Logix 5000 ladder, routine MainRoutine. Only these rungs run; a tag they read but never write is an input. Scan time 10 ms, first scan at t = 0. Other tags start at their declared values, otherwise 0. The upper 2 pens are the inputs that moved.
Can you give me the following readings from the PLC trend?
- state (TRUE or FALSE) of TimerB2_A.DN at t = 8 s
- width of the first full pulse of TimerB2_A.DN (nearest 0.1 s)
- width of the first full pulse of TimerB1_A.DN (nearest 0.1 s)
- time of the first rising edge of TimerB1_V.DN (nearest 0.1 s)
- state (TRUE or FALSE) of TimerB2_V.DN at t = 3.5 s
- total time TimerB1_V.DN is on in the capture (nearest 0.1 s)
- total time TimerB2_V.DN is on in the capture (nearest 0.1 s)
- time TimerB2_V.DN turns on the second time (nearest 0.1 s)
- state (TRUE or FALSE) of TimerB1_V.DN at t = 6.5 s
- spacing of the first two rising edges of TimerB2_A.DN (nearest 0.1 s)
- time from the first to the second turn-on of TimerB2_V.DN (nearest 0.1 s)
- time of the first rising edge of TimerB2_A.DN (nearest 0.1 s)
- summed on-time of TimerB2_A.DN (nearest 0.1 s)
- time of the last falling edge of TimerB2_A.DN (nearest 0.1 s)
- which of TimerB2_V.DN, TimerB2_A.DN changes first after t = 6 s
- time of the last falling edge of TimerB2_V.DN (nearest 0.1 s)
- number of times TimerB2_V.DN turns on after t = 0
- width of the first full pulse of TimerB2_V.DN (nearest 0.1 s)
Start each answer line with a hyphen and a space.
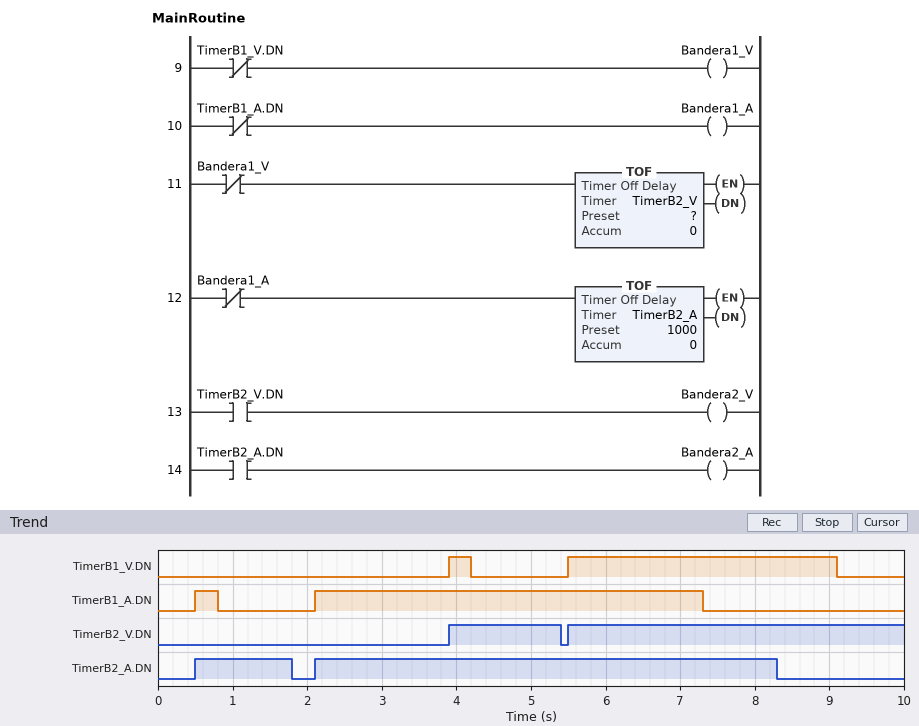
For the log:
- TRUE
- 1.3 s
- 0.3 s
- 3.9 s
- FALSE
- 3.9 s
- 6.0 s
- 5.5 s
- TRUE
- 1.6 s
- 1.6 s
- 0.5 s
- 7.5 s
- 8.3 s
- TimerB2_A.DN
- 5.4 s
- 2
- 1.5 s
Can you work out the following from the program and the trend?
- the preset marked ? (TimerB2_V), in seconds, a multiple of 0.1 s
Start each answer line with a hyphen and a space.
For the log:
- 1.2 s
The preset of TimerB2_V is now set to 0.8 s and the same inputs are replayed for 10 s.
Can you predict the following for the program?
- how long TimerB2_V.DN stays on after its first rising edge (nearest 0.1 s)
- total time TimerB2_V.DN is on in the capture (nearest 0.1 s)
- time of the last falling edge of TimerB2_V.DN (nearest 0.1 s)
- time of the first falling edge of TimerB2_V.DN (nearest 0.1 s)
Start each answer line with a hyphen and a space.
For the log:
- 1.1 s
- 5.5 s
- 9.9 s
- 5.0 s
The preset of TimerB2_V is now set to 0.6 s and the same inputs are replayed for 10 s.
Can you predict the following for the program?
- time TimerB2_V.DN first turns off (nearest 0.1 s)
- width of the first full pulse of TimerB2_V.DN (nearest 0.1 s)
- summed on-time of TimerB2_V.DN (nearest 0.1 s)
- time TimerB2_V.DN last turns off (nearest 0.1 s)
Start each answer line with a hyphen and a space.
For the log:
- 4.8 s
- 0.9 s
- 5.1 s
- 9.7 s
